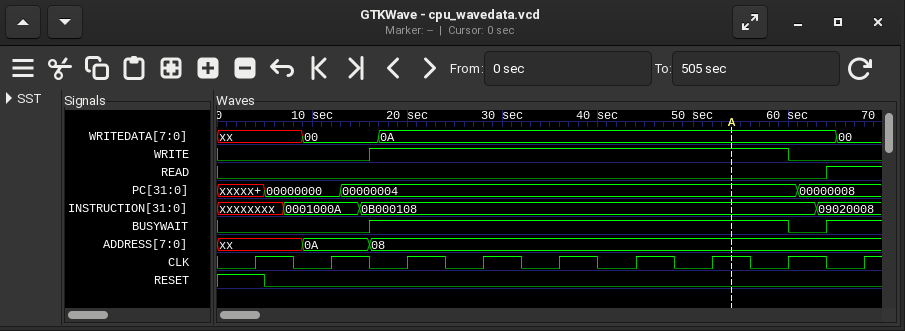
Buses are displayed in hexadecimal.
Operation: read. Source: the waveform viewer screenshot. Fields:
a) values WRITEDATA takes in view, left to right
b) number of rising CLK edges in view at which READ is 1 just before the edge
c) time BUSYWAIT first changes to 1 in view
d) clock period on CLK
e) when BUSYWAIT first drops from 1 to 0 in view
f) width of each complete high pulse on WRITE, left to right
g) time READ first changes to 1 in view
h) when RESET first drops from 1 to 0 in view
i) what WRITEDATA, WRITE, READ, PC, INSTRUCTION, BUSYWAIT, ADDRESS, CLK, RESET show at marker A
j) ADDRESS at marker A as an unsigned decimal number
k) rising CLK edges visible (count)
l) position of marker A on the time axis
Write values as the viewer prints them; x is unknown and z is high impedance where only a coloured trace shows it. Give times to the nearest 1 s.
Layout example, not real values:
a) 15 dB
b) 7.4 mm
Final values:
a) xx, 00, 0A, 00
b) 1
c) 16 s
d) 8 s
e) 60 s
f) 44 s
g) 64 s
h) 5 s
i) WRITEDATA=0A, WRITE=1, READ=0, PC=00000004, INSTRUCTION=0B000108, BUSYWAIT=1, ADDRESS=08, CLK=1, RESET=0
j) 8
k) 9
l) 54 s
